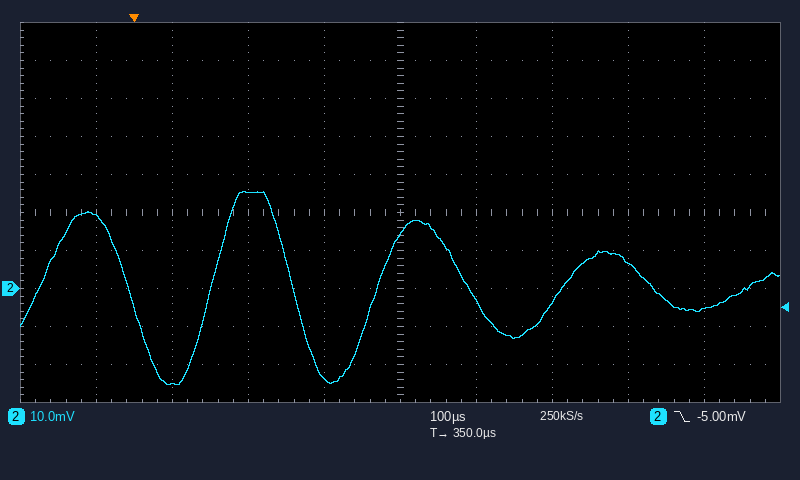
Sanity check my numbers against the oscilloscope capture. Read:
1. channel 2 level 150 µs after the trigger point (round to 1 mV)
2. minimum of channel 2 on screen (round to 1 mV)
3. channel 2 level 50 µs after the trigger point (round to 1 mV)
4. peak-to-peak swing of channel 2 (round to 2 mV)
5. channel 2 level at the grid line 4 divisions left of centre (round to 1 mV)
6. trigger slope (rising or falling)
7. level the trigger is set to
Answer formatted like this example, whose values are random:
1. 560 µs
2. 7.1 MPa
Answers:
1. 25 mV
2. -25 mV
3. -25 mV
4. 50 mV
5. 19 mV
6. falling
7. -5.00 mV
